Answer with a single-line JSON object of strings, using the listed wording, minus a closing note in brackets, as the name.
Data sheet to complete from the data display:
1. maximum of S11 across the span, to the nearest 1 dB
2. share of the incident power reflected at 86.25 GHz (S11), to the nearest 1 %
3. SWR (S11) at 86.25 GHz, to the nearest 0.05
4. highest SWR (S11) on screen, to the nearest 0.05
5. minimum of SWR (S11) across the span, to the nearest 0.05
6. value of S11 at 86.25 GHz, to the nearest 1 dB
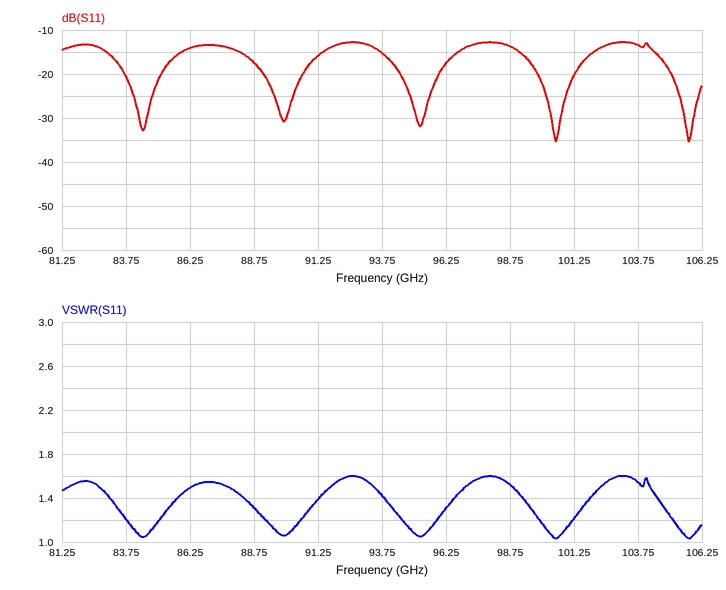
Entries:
{"maximum of S11 across the span, to the nearest 1 dB": "-13 dB", "share of the incident power reflected at 86.25 GHz (S11), to the nearest 1 %": "4 %", "SWR (S11) at 86.25 GHz, to the nearest 0.05": "1.50", "highest SWR (S11) on screen, to the nearest 0.05": "1.60", "minimum of SWR (S11) across the span, to the nearest 0.05": "1.05", "value of S11 at 86.25 GHz, to the nearest 1 dB": "-14 dB"}
